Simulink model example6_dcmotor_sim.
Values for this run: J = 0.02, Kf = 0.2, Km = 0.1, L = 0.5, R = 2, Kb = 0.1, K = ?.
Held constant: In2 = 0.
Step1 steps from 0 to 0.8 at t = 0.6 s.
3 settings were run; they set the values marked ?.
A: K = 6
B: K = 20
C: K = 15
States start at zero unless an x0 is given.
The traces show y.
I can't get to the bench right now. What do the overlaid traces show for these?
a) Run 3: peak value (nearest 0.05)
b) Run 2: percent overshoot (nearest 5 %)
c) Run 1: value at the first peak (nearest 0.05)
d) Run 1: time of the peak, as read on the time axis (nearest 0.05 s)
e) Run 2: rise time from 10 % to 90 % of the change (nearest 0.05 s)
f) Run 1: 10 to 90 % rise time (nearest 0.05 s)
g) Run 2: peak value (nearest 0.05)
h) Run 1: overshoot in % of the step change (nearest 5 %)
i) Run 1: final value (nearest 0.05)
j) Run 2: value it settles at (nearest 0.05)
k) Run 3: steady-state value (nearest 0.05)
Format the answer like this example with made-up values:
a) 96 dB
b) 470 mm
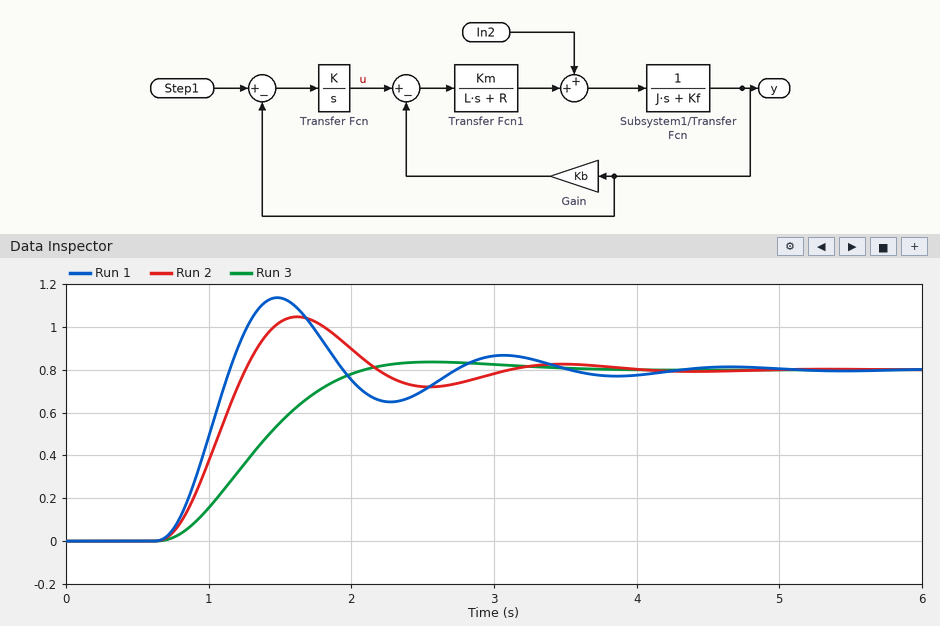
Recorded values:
a) 0.85
b) 30 %
c) 1.15
d) 1.50 s
e) 0.40 s
f) 0.35 s
g) 1.05
h) 40 %
i) 0.80
j) 0.80
k) 0.80
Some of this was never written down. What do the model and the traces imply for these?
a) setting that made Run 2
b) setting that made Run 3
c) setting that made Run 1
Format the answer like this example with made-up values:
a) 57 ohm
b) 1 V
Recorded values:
a) C
b) A
c) B
